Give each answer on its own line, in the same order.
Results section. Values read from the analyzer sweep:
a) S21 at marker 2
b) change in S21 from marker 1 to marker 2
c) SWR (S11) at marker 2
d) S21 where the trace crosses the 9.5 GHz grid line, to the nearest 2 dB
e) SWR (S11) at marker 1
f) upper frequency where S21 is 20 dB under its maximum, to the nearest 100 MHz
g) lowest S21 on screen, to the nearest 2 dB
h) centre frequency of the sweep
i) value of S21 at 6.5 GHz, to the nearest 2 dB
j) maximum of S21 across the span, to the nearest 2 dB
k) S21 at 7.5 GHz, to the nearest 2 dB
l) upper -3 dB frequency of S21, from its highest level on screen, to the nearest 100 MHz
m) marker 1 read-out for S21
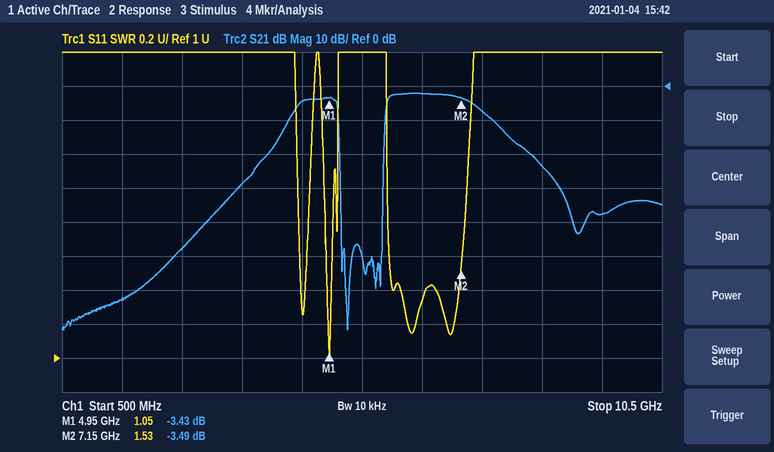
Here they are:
-3.49 dB
-0.06 dB
1.53
-38 dB
1.05
8.4 GHz
-72 dB
5.5 GHz
-2 dB
-2 dB
-8 dB
7.3 GHz
-3.43 dB
